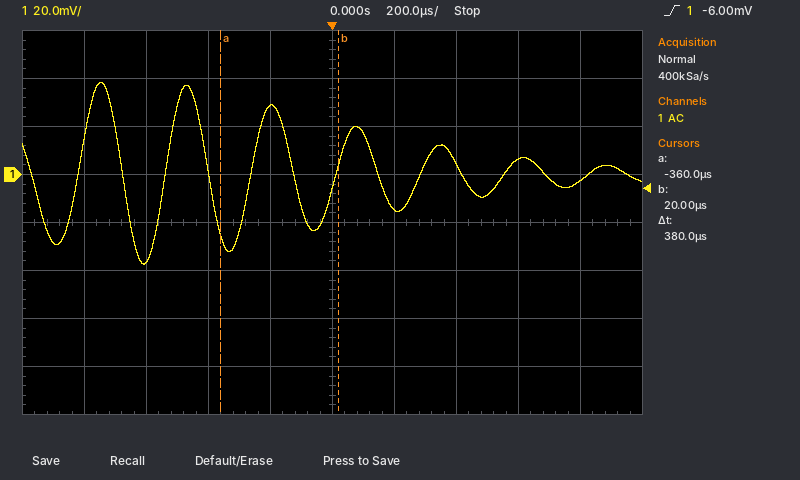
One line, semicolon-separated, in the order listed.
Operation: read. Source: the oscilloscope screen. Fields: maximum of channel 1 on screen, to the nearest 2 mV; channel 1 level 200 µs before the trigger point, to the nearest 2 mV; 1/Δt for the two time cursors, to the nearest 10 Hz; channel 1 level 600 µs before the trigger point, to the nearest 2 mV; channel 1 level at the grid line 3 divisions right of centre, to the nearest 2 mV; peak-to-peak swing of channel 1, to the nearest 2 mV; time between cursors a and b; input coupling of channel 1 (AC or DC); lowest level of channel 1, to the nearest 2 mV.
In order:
38 mV; 28 mV; 2.63 kHz; -36 mV; 6 mV; 76 mV; 380 µs; AC; -38 mV
